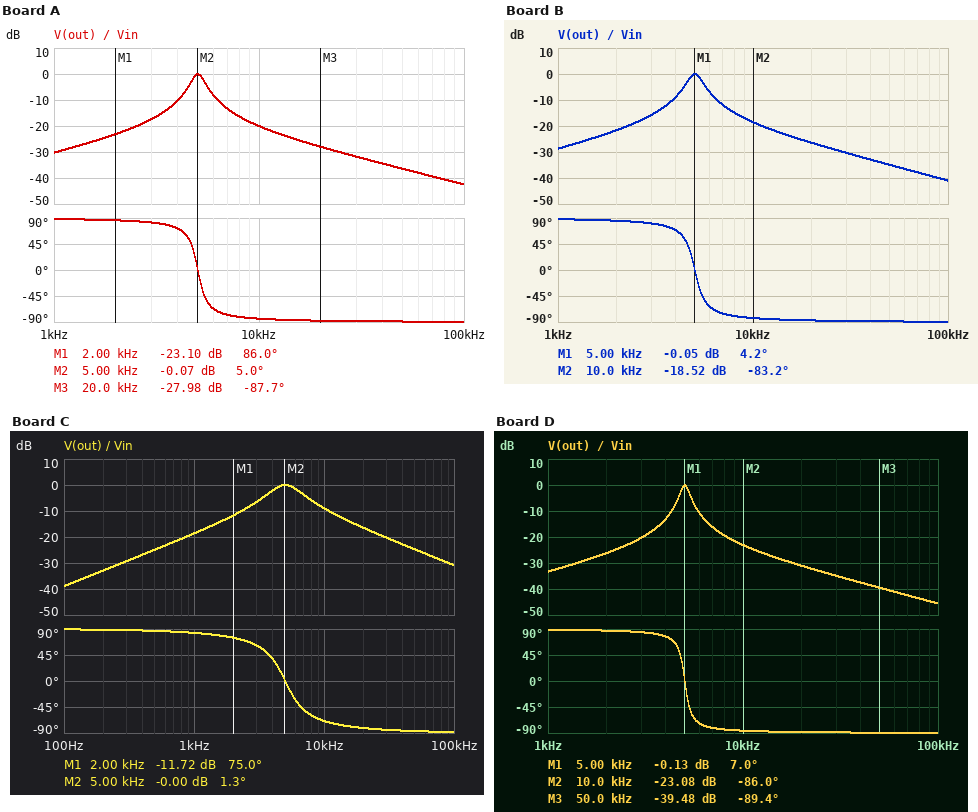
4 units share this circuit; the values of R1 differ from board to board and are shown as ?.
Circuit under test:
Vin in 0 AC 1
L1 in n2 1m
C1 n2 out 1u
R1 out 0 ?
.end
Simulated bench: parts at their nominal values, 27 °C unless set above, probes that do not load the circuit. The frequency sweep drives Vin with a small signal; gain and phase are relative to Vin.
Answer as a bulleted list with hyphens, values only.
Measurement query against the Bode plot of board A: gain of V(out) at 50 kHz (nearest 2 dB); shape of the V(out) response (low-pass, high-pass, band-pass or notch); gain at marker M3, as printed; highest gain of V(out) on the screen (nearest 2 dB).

- -36 dB
- band-pass
- -27.98 dB
- 0 dB
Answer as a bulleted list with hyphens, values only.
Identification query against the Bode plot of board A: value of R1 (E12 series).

- 4.7 Ω
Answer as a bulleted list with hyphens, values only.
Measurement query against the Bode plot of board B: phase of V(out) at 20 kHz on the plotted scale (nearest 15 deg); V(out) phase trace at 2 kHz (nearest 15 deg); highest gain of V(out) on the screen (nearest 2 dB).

- -90 deg
- 90 deg
- 0 dB
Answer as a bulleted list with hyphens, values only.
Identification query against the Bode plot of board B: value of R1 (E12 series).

- 5.6 Ω
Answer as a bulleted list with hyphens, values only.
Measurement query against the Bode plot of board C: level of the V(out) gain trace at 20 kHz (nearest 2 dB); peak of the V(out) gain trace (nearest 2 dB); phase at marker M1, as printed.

- -16 dB
- 0 dB
- 75.0 deg
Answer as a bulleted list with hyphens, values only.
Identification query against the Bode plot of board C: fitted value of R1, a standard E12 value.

- 18 Ω
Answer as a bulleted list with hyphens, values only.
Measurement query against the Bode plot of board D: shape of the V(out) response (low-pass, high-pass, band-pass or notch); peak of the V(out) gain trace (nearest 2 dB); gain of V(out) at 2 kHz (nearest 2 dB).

- band-pass
- 0 dB
- -26 dB
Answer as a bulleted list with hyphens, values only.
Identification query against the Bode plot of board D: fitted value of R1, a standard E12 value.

- 3.3 Ω
